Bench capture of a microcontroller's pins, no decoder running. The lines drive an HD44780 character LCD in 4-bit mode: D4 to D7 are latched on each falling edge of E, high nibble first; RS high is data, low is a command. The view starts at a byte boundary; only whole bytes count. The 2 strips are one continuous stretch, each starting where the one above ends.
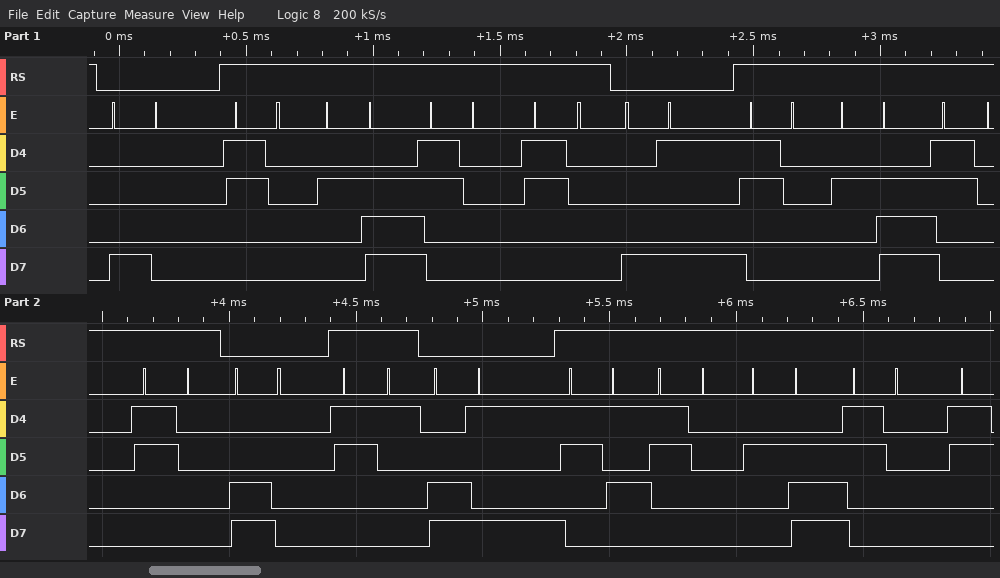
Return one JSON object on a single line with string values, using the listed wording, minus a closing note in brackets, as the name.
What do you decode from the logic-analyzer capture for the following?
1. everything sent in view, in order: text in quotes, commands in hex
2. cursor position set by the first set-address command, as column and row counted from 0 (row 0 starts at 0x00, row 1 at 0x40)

{"everything sent in view, in order: text in quotes, commands in hex": "0x80 \"0.00\" 0x89 \"0.00\" 0xC0 \"1\" 0xC9 \"50.0\"", "cursor position set by the first set-address command, as column and row counted from 0": "column 0, row 0"}
